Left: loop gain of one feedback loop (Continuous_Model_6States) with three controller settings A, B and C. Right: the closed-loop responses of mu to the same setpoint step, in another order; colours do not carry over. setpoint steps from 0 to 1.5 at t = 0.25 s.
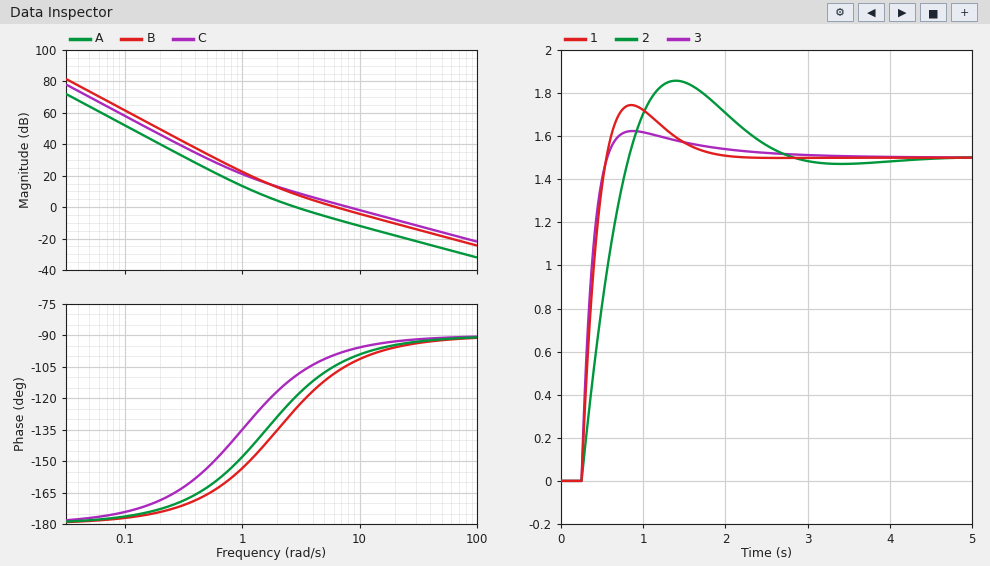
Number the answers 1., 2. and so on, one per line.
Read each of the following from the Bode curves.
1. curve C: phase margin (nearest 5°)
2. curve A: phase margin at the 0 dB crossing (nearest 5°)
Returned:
1. 85°
2. 60°
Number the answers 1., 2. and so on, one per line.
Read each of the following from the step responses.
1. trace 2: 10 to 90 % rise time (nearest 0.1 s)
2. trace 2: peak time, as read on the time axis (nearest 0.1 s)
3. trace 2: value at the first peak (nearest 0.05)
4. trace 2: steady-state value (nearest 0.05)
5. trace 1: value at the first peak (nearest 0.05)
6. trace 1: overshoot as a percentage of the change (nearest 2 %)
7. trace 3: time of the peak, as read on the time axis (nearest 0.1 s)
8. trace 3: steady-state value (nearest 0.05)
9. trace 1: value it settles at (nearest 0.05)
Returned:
1. 0.4 s
2. 1.4 s
3. 1.85
4. 1.50
5. 1.75
6. 16 %
7. 0.9 s
8. 1.50
9. 1.50
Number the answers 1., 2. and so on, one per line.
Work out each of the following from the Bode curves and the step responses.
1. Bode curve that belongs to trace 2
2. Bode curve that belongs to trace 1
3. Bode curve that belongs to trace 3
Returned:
1. A
2. B
3. C
